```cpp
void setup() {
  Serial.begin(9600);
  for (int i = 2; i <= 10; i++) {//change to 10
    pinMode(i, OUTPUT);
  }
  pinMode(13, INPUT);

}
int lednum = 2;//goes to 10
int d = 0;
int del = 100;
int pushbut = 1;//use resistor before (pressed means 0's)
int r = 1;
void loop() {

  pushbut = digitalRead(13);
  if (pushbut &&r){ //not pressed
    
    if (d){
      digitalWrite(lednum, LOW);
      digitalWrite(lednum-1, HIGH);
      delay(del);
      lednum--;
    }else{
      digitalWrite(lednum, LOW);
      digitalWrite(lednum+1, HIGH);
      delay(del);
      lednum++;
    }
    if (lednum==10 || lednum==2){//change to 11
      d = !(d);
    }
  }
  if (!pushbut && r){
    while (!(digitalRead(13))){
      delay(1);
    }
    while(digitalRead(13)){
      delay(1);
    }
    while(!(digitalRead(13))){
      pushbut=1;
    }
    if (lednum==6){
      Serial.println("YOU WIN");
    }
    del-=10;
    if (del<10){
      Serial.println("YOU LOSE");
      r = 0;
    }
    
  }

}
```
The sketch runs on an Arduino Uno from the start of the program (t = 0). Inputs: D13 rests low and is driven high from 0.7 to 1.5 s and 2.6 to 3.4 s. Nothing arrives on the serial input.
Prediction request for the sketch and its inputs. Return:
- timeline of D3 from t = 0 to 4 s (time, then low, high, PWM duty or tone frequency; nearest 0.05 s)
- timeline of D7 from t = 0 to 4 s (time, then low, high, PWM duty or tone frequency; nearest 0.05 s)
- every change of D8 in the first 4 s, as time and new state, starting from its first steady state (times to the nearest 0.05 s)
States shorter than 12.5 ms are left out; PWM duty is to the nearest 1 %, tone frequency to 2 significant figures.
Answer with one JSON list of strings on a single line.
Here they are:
["0 s low; 2.6 s high; 2.7 s low", "0 s low; 2.95 s high; 3.05 s low", "0 s low; 3.05 s high; 3.15 s low"]
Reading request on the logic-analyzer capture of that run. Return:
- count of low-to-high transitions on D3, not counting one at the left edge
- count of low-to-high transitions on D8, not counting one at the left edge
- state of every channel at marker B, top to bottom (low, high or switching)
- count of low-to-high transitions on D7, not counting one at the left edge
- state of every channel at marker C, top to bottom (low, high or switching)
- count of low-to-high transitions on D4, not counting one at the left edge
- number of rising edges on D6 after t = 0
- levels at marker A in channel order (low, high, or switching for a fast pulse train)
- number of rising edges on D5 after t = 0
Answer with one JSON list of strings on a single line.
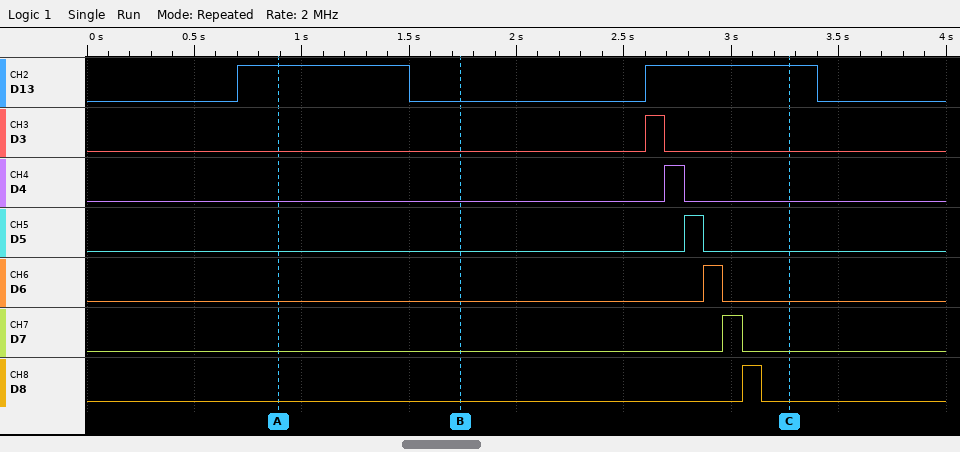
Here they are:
["1", "1", "D13 low, D3 low, D4 low, D5 low, D6 low, D7 low, D8 low", "1", "D13 high, D3 low, D4 low, D5 low, D6 low, D7 low, D8 low", "1", "1", "D13 high, D3 low, D4 low, D5 low, D6 low, D7 low, D8 low", "1"]
